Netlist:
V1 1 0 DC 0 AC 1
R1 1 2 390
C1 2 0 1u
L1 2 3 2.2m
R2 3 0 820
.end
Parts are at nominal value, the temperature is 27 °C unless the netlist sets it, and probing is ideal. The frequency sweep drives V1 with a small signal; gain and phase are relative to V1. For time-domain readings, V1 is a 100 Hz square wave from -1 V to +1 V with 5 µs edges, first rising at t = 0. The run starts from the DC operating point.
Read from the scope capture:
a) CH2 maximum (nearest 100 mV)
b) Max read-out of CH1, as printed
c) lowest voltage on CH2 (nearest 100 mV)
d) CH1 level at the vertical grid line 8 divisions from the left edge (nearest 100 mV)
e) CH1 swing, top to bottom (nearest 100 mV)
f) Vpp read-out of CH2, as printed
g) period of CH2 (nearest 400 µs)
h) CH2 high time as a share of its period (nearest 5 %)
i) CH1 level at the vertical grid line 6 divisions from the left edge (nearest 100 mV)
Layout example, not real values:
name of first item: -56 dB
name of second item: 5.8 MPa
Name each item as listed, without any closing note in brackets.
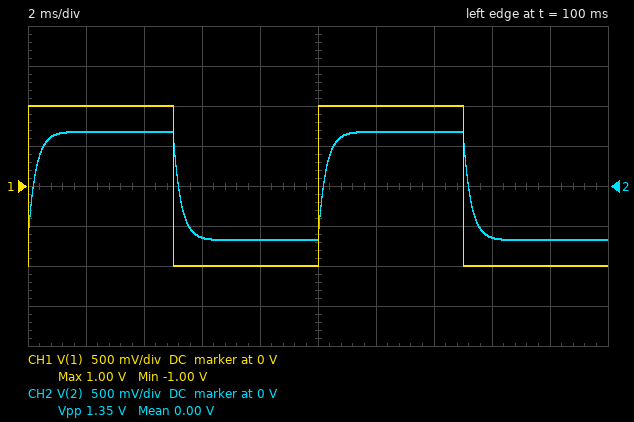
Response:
CH2 maximum: 700 mV
Max read-out of CH1, as printed: 1.00 V
lowest voltage on CH2: -700 mV
CH1 level at the vertical grid line 8 divisions from the left edge: -1.0 V
CH1 swing, top to bottom: 2.0 V
Vpp read-out of CH2, as printed: 1.35 V
period of CH2: 10.0 ms
CH2 high time as a share of its period: 50 %
CH1 level at the vertical grid line 6 divisions from the left edge: 1.0 V
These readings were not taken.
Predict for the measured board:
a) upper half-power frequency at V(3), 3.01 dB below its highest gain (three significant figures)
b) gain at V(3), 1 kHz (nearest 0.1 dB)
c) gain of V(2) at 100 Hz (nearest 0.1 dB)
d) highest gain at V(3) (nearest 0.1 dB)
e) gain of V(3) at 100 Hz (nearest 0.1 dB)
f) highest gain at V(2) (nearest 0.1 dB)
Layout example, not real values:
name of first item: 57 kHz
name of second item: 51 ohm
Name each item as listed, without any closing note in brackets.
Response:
upper half-power frequency at V(3), 3.01 dB below its highest gain: 604 Hz
gain at V(3), 1 kHz: -9.1 dB
gain of V(2) at 100 Hz: -3.5 dB
highest gain at V(3): -3.4 dB
gain of V(3) at 100 Hz: -3.5 dB
highest gain at V(2): -3.4 dB
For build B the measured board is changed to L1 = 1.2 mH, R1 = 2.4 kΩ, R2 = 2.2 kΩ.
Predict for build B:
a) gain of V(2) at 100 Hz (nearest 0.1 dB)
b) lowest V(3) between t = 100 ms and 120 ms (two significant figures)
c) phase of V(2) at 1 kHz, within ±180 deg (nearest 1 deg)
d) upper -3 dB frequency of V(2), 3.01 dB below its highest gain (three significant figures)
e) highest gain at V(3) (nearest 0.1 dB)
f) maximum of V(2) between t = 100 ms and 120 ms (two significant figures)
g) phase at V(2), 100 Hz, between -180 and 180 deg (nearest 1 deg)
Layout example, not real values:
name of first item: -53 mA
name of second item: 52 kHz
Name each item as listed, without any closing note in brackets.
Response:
gain of V(2) at 100 Hz: -8.2 dB
lowest V(3) between t = 100 ms and 120 ms: -470 mV
phase of V(2) at 1 kHz, within ±180 deg: -82 deg
upper -3 dB frequency of V(2), 3.01 dB below its highest gain: 139 Hz
highest gain at V(3): -6.4 dB
maximum of V(2) between t = 100 ms and 120 ms: 470 mV
phase at V(2), 100 Hz, between -180 and 180 deg: -36 deg
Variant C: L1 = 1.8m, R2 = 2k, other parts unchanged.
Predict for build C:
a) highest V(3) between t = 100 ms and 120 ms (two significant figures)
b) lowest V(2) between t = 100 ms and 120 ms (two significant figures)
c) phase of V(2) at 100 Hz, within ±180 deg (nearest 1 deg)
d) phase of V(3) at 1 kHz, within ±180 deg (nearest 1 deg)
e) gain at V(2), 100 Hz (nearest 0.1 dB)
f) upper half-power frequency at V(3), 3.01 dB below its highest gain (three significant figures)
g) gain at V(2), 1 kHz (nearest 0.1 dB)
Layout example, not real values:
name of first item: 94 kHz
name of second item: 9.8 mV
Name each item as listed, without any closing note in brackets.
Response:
highest V(3) between t = 100 ms and 120 ms: 840 mV
lowest V(2) between t = 100 ms and 120 ms: -840 mV
phase of V(2) at 100 Hz, within ±180 deg: -12 deg
phase of V(3) at 1 kHz, within ±180 deg: -64 deg
gain at V(2), 100 Hz: -1.7 dB
upper half-power frequency at V(3), 3.01 dB below its highest gain: 488 Hz
gain at V(2), 1 kHz: -8.7 dB
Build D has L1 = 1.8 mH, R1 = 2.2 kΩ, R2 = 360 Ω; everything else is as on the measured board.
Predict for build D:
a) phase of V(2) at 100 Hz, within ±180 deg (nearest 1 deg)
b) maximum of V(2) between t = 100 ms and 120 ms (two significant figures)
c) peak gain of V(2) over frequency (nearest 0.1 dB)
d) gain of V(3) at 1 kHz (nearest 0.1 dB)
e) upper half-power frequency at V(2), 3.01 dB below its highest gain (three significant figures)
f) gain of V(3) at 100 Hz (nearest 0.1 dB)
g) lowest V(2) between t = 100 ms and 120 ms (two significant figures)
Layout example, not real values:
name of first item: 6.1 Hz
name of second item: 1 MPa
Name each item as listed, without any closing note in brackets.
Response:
phase of V(2) at 100 Hz, within ±180 deg: -11 deg
maximum of V(2) between t = 100 ms and 120 ms: 140 mV
peak gain of V(2) over frequency: -17.0 dB
gain of V(3) at 1 kHz: -23.7 dB
upper half-power frequency at V(2), 3.01 dB below its highest gain: 522 Hz
gain of V(3) at 100 Hz: -17.2 dB
lowest V(2) between t = 100 ms and 120 ms: -140 mV
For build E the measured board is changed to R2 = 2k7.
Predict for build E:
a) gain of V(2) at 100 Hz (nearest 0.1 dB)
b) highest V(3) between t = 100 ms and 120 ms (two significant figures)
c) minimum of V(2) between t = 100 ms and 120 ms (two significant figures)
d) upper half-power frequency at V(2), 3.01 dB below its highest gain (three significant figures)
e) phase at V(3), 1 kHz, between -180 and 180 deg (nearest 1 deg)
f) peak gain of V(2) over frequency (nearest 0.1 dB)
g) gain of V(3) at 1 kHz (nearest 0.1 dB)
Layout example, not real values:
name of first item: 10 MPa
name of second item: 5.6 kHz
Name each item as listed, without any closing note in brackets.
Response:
gain of V(2) at 100 Hz: -1.4 dB
highest V(3) between t = 100 ms and 120 ms: 870 mV
minimum of V(2) between t = 100 ms and 120 ms: -870 mV
upper half-power frequency at V(2), 3.01 dB below its highest gain: 467 Hz
phase at V(3), 1 kHz, between -180 and 180 deg: -65 deg
peak gain of V(2) over frequency: -1.2 dB
gain of V(3) at 1 kHz: -8.6 dB
